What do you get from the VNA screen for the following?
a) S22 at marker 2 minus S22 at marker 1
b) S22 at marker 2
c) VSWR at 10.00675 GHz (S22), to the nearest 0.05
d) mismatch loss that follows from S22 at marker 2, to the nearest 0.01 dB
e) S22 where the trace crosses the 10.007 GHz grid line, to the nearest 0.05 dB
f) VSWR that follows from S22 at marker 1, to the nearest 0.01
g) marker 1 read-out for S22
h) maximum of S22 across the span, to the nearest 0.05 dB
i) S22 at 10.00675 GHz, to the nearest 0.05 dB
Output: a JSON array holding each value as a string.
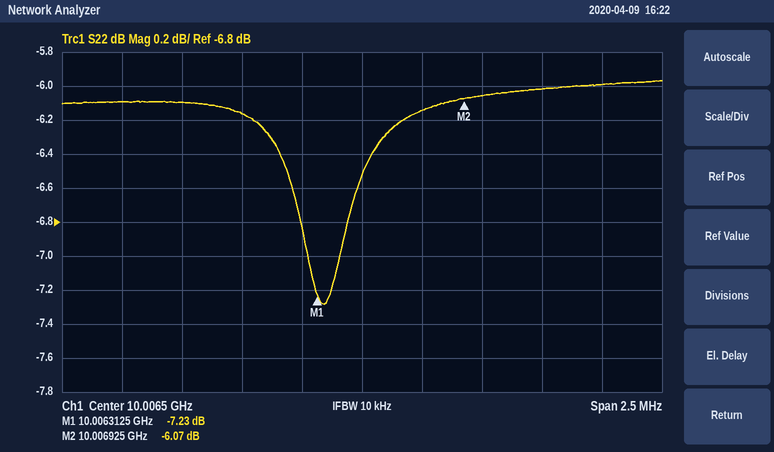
["1.16 dB", "-6.07 dB", "2.95", "1.23 dB", "-6.05 dB", "2.54", "-7.23 dB", "-5.95 dB", "-6.15 dB"]
